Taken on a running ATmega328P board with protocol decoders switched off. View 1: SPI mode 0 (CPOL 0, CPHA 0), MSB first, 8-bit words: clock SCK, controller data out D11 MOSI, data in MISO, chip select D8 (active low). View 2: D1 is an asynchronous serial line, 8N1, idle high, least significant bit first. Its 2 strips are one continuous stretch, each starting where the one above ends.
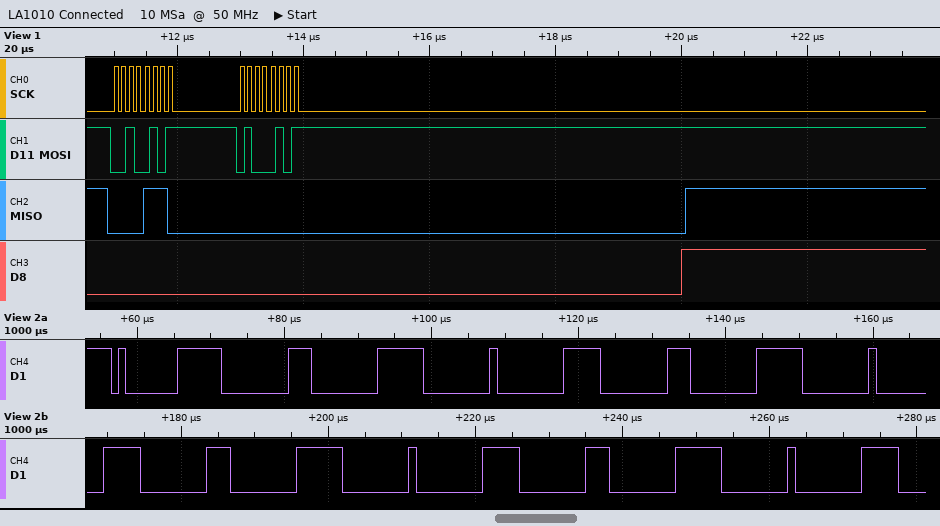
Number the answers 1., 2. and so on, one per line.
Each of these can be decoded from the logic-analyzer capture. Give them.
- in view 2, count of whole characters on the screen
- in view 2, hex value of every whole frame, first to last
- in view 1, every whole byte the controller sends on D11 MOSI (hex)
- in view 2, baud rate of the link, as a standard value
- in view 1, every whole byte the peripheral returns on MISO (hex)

1. 17
2. 01 00 00 00 00 00 00 00 00 00 00 00 00 00 00 00 00
3. 25 45
4. 1000000 baud
5. 0E 00
